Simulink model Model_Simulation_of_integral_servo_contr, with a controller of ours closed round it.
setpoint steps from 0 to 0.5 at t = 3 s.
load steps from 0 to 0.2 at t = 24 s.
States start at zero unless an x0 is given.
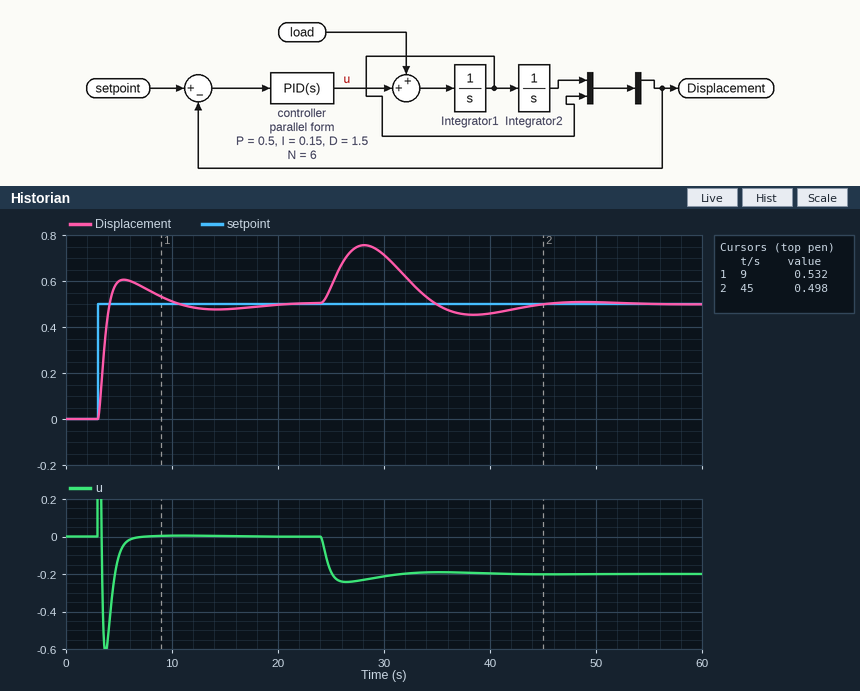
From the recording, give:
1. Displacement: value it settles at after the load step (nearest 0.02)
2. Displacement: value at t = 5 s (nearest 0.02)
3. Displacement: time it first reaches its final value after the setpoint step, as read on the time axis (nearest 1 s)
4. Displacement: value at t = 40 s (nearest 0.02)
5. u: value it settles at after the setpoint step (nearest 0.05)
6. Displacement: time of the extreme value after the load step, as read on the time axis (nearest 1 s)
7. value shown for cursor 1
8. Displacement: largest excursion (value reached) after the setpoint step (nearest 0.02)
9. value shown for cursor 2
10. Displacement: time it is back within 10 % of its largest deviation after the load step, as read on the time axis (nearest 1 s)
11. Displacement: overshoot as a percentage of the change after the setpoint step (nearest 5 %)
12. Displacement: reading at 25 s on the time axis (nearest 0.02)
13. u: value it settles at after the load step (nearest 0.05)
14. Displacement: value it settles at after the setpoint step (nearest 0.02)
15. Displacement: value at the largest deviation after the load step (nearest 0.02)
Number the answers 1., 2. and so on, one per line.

1. 0.50
2. 0.60
3. 4 s
4. 0.46
5. 0.00
6. 28 s
7. 0.532
8. 0.60
9. 0.498
10. 42 s
11. 20 %
12. 0.58
13. -0.20
14. 0.50
15. 0.76
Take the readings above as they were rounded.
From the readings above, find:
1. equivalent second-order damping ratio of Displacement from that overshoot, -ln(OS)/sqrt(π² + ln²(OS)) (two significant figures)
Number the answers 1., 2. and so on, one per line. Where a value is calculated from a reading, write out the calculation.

1. ln(0.2) = -1.609; 1.609 / sqrt(9.870 + 2.590) = 0.46
